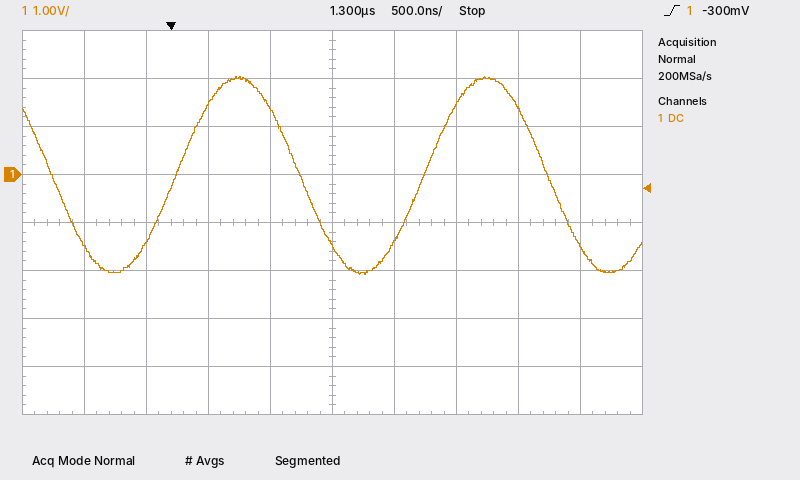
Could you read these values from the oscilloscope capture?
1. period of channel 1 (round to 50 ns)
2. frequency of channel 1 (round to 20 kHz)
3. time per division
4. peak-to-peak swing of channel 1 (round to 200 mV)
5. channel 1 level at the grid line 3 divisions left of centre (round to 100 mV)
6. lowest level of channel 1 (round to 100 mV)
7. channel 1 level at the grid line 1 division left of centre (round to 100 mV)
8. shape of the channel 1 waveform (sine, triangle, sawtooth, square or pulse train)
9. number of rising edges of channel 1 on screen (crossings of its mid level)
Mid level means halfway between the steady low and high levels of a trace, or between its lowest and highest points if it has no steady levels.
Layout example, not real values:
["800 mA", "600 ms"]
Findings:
["2.00 µs", "500 kHz", "500 ns", "4.2 V", "-1.4 V", "-2.1 V", "1.4 V", "sine", "2"]
